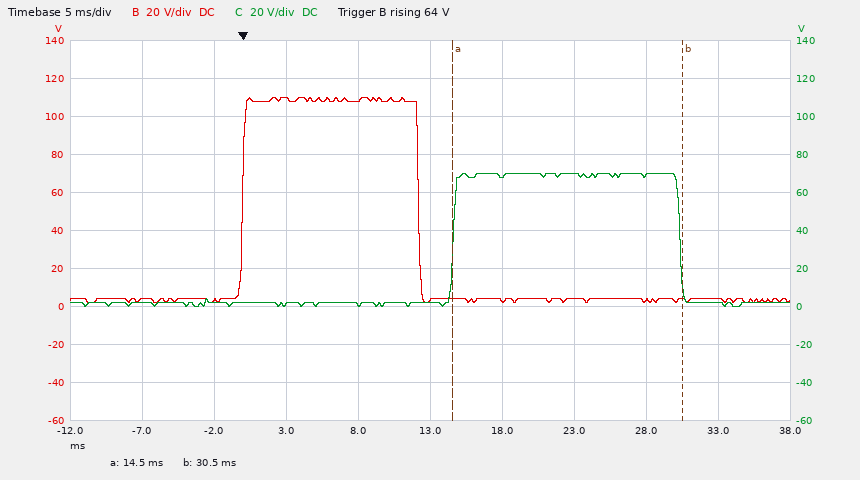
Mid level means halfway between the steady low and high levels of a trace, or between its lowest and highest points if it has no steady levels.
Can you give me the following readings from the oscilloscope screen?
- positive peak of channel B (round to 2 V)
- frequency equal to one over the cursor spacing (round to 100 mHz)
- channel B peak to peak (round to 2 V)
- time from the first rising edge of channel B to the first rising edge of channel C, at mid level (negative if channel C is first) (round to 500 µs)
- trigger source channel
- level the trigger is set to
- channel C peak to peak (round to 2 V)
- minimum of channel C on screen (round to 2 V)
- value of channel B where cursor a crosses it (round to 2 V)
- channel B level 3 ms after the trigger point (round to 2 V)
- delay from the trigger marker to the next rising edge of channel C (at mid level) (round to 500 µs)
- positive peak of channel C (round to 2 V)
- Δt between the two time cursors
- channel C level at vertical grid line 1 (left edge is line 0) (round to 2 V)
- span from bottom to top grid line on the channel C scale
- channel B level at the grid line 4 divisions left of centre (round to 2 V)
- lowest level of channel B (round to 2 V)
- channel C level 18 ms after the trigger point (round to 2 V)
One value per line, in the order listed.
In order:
110 V
62.5 Hz
108 V
+14.5 ms
channel B
64 V
70 V
0 V
4 V
110 V
14.5 ms
70 V
16.0 ms
2 V
200 V
4 V
2 V
68 V
